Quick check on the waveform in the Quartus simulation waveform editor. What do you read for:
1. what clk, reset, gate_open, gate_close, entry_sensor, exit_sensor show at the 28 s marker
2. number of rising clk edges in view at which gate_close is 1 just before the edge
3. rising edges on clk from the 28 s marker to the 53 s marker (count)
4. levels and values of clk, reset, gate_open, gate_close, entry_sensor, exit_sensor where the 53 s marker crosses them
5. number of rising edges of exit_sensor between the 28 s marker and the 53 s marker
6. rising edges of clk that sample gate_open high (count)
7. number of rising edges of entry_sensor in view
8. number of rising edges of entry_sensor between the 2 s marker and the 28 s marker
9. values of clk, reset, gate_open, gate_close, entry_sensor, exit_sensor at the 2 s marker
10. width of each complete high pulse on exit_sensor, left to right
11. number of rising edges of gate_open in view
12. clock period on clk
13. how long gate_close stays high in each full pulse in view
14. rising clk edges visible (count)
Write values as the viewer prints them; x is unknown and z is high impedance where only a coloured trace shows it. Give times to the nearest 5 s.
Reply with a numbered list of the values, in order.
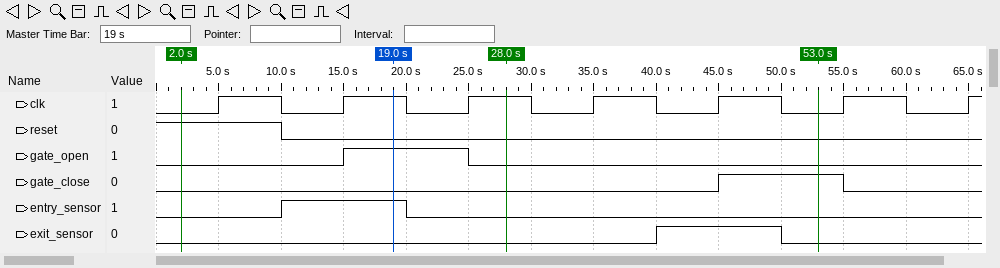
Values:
1. clk=1, reset=0, gate_open=0, gate_close=0, entry_sensor=0, exit_sensor=0
2. 1
3. 2
4. clk=0, reset=0, gate_open=0, gate_close=1, entry_sensor=0, exit_sensor=0
5. 1
6. 1
7. 1
8. 1
9. clk=0, reset=1, gate_open=0, gate_close=0, entry_sensor=0, exit_sensor=0
10. 10 s
11. 1
12. 10 s
13. 10 s
14. 7
